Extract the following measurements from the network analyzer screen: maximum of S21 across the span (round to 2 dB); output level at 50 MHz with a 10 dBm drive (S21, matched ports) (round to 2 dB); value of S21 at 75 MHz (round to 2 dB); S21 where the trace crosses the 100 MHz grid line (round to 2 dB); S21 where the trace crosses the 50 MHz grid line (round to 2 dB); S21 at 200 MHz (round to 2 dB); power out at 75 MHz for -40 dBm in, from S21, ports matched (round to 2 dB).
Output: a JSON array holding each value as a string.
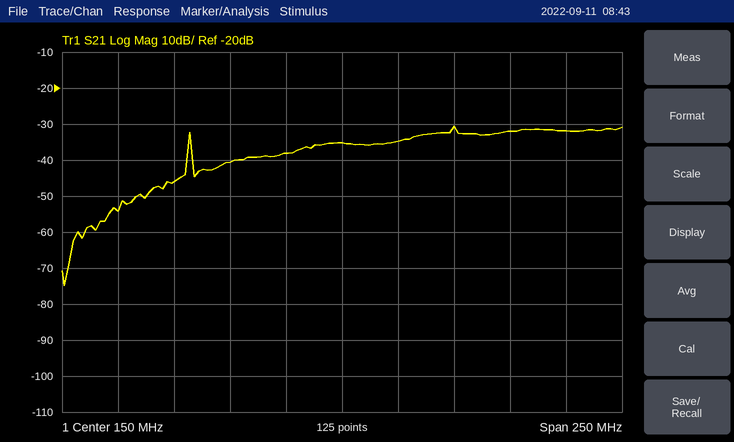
["-30 dB", "-44 dBm", "-46 dB", "-40 dB", "-54 dB", "-30 dB", "-86 dBm"]
